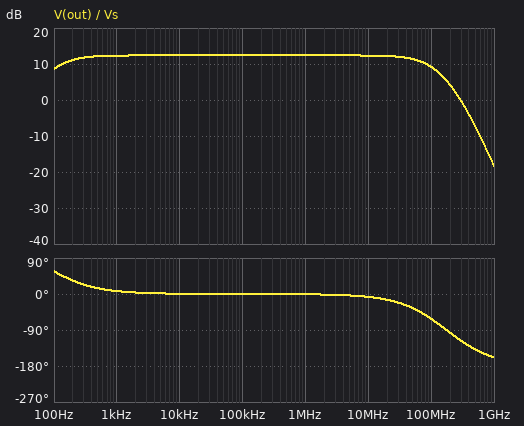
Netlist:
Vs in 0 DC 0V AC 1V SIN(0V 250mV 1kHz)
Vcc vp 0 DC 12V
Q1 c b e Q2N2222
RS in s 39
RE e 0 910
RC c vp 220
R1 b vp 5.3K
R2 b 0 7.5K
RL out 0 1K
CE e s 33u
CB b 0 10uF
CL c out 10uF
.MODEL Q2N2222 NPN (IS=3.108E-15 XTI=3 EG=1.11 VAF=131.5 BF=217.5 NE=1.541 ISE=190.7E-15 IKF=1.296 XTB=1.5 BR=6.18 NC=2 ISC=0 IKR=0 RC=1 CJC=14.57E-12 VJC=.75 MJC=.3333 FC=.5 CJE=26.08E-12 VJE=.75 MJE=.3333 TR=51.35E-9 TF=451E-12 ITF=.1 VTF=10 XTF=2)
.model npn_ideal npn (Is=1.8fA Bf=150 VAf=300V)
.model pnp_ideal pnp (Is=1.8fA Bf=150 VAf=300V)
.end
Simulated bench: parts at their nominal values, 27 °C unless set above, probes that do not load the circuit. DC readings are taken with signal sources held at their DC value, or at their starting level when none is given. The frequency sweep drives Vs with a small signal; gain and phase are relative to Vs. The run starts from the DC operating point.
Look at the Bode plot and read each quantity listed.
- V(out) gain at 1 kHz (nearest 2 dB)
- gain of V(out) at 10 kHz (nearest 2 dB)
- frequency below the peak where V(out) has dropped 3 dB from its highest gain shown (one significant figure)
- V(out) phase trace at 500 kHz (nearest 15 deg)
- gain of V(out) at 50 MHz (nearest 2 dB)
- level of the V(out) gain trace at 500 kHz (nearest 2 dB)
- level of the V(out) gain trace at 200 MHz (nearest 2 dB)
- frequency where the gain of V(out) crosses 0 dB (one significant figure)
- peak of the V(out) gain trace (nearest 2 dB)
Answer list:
12 dB
12 dB
100 Hz
0 deg
12 dB
12 dB
4 dB
300 MHz
12 dB
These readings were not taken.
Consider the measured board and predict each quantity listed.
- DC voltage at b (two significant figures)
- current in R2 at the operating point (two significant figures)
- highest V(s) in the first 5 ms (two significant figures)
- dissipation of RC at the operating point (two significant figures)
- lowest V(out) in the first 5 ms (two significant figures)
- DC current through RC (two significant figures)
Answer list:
6.9 V
920 µA
62 mV
9.9 mW
-1.1 V
6.7 mA
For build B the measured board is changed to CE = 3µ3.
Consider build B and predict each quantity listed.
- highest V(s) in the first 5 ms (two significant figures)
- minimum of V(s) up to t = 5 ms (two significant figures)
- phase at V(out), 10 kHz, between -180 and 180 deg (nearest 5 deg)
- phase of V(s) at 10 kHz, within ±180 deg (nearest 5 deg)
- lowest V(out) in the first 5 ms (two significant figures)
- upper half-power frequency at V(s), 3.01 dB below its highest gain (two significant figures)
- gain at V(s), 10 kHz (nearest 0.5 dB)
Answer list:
200 mV
-190 mV
5 deg
-45 deg
-700 mV
1.1 kHz
-17.0 dB
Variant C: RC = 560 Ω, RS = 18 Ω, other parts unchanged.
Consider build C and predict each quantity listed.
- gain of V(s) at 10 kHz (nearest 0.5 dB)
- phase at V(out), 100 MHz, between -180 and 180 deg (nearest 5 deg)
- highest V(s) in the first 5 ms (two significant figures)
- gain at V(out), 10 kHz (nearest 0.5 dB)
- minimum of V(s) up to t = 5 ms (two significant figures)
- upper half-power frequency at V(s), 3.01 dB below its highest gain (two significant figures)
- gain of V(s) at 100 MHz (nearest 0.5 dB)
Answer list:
-15.0 dB
-85 deg
130 mV
24.0 dB
-110 mV
230 Hz
-15.5 dB
